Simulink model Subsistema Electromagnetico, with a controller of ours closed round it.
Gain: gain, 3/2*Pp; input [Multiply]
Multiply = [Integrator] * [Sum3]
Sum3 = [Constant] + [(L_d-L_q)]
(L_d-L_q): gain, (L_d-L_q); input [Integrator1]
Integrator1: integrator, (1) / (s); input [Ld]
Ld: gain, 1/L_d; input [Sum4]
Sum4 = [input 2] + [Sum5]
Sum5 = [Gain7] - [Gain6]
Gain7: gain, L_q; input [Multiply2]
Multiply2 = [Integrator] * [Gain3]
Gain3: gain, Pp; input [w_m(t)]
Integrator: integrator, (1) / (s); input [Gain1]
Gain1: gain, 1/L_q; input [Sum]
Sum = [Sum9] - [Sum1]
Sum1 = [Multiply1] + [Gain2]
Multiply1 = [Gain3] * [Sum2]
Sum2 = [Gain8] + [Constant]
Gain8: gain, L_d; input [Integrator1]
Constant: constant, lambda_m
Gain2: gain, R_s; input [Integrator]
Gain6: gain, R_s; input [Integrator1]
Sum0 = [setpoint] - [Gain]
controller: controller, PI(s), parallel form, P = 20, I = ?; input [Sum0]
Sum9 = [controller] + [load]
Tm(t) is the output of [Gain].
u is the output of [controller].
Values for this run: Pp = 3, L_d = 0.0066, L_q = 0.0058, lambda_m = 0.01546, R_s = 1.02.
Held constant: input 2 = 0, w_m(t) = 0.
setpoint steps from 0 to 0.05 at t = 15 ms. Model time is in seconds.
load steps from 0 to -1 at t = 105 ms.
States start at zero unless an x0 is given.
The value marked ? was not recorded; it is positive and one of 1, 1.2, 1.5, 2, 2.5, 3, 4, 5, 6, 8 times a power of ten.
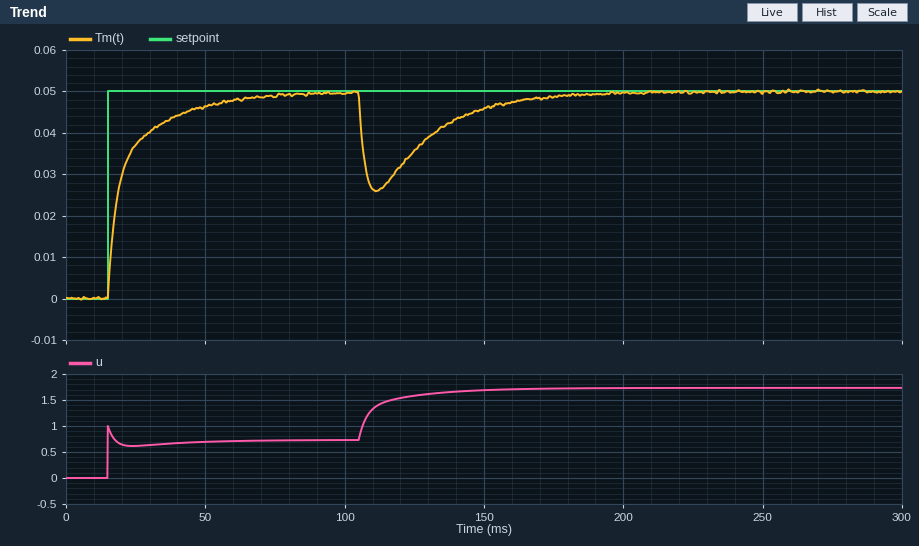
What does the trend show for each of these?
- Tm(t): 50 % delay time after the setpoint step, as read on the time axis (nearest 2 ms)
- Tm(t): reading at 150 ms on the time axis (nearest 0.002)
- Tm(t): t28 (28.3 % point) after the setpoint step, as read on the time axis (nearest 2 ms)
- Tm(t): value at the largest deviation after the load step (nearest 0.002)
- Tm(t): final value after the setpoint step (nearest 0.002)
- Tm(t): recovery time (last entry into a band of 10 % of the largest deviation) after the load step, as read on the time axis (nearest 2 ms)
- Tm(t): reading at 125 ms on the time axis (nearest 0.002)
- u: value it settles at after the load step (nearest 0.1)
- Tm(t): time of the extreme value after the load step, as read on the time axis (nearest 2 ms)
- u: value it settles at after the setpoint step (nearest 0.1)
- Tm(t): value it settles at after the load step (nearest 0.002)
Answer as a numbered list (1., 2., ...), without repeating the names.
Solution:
1. 18 ms
2. 0.046
3. 16 ms
4. 0.026
5. 0.050
6. 162 ms
7. 0.036
8. 1.7
9. 112 ms
10. 0.7
11. 0.050
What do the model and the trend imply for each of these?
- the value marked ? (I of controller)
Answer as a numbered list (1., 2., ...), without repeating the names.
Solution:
1. 1500
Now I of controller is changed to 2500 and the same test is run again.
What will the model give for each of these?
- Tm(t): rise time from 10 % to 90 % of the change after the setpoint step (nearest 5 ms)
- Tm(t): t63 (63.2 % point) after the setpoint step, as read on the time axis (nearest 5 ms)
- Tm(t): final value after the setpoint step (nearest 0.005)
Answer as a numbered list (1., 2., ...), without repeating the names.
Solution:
1. 15 ms
2. 20 ms
3. 0.050
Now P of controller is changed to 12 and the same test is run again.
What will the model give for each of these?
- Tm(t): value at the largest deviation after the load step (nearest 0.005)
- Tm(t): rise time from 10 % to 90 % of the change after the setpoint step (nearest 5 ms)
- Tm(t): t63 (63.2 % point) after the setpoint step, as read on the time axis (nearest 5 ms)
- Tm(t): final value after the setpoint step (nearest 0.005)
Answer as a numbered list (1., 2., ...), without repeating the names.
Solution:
1. 0.020
2. 25 ms
3. 25 ms
4. 0.050
